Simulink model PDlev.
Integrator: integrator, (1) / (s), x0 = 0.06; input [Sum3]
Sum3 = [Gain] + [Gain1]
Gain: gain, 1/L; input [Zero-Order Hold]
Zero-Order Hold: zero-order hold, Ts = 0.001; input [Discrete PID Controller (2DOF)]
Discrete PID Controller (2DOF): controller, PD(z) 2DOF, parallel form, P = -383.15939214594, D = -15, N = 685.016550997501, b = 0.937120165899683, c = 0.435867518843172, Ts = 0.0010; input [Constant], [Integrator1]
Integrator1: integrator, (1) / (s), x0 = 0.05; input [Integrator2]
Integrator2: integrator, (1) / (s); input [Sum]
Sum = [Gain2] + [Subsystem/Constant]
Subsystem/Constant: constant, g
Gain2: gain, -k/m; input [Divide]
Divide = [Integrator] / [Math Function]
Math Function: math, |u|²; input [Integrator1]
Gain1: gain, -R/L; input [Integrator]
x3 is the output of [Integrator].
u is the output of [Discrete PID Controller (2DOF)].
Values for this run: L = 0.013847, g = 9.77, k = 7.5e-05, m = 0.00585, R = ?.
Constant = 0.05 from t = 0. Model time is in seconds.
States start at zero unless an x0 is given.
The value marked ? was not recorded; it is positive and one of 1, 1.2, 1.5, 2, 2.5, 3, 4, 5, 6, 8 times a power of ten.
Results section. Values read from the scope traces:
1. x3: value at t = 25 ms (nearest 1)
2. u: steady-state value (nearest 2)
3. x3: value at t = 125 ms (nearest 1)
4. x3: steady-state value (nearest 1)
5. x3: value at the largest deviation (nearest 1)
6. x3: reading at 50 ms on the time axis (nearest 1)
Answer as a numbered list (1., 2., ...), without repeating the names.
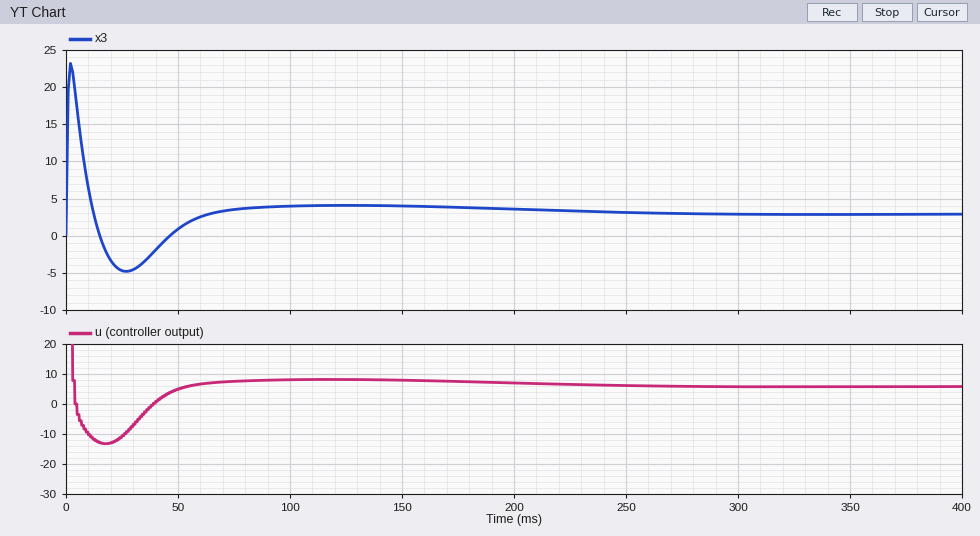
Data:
1. -5
2. 6
3. 4
4. 3
5. 23
6. 1
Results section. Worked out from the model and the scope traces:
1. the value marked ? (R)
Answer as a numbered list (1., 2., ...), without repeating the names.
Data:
1. 2
